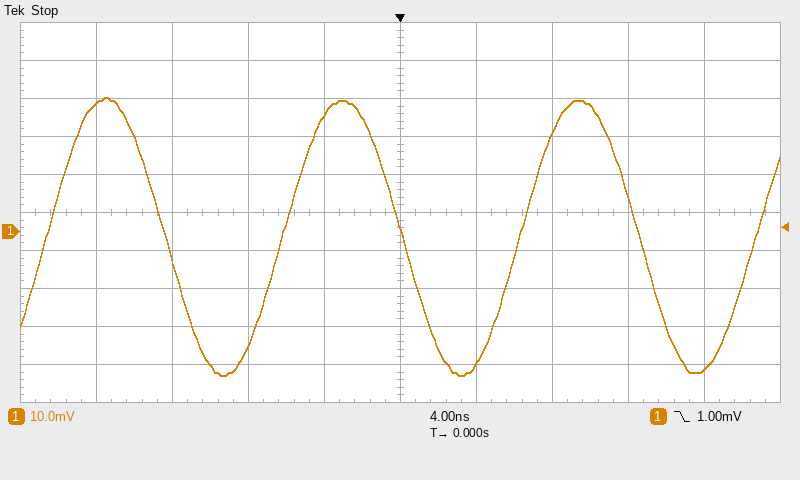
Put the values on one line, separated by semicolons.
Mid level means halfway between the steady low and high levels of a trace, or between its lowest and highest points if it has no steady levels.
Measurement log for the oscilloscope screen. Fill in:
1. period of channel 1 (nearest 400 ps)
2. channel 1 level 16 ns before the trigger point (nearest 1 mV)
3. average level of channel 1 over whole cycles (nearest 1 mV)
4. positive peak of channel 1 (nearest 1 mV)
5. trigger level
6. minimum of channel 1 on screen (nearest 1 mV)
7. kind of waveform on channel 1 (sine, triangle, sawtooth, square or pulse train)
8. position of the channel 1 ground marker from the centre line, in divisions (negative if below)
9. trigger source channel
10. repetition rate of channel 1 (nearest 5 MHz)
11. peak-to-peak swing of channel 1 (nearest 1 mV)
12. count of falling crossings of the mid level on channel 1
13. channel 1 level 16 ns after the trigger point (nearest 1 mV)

12.4 ns; 34 mV; -1 mV; 35 mV; 1.00 mV; -38 mV; sine; -0.5 div; channel 1; 80 MHz; 73 mV; 3; -36 mV
